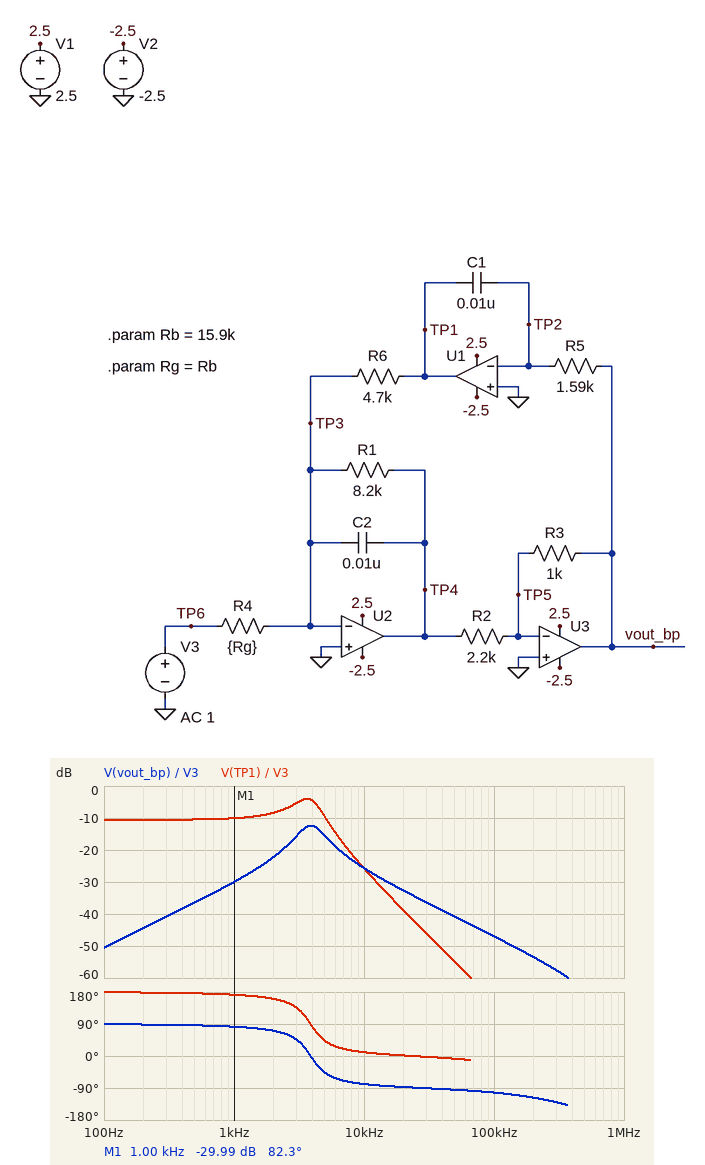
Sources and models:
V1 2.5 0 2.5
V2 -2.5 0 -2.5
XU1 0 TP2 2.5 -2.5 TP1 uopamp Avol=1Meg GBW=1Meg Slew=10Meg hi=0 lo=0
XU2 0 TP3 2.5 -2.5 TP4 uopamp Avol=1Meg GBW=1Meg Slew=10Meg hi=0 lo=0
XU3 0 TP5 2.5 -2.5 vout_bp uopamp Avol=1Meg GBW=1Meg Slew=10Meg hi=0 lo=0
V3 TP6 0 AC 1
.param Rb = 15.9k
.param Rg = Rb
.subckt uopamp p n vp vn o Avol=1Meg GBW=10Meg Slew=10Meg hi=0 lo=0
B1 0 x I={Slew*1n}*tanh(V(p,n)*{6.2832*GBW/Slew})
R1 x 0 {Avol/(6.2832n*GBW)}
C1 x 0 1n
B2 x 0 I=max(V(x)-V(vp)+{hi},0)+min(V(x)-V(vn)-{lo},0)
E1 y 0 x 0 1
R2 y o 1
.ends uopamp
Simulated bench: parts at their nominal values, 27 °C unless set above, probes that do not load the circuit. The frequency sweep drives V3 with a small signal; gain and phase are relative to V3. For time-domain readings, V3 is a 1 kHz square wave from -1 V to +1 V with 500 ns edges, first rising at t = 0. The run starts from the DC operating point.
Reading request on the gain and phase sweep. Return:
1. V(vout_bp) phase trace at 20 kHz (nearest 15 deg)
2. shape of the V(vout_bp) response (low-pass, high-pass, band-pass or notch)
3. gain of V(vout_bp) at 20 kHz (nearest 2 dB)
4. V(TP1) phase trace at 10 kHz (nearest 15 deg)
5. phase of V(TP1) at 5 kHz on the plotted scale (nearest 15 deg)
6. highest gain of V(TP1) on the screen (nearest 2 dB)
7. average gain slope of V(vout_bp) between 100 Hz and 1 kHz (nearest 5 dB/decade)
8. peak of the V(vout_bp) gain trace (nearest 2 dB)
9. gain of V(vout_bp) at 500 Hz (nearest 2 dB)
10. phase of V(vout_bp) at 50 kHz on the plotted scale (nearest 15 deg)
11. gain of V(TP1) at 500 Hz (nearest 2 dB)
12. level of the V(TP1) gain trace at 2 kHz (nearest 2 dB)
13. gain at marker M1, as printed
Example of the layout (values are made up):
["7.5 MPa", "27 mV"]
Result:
["-90 deg", "band-pass", "-32 dB", "15 deg", "45 deg", "-4 dB", "20 dB/decade", "-12 dB", "-36 dB", "-90 deg", "-10 dB", "-8 dB", "-29.99 dB"]
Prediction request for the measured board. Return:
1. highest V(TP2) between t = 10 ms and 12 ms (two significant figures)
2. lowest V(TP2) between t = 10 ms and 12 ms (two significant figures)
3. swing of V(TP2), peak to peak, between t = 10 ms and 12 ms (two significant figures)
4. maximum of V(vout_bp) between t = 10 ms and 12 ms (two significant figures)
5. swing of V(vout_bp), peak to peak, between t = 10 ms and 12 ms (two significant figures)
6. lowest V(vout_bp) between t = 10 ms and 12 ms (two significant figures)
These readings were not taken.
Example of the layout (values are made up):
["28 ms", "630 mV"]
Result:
["1.6 mV", "-1.6 mV", "3.2 mV", "160 mV", "320 mV", "-160 mV"]
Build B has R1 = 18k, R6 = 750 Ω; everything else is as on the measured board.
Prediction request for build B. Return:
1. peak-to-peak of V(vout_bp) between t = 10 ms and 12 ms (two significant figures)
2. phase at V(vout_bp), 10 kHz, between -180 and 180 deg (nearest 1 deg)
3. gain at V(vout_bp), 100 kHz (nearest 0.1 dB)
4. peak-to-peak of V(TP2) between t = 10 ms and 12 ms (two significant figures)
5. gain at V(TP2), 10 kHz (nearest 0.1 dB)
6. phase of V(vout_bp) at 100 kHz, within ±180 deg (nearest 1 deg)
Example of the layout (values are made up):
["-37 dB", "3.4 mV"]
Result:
["140 mV", "-52 deg", "-47.1 dB", "1.4 mV", "-45.7 dB", "-104 deg"]
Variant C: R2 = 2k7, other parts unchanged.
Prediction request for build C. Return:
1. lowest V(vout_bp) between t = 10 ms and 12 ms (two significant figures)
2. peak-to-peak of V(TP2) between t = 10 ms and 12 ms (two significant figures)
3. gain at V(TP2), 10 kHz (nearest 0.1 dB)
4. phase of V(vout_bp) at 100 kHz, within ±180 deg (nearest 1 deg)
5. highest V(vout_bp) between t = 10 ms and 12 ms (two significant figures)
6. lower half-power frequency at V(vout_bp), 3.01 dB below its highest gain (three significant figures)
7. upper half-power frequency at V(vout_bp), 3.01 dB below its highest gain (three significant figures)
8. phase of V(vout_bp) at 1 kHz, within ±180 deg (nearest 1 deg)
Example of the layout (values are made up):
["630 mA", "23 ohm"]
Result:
["-150 mV", "3.0 mV", "-67.8 dB", "-102 deg", "150 mV", "2.70 kHz", "4.59 kHz", "80 deg"]
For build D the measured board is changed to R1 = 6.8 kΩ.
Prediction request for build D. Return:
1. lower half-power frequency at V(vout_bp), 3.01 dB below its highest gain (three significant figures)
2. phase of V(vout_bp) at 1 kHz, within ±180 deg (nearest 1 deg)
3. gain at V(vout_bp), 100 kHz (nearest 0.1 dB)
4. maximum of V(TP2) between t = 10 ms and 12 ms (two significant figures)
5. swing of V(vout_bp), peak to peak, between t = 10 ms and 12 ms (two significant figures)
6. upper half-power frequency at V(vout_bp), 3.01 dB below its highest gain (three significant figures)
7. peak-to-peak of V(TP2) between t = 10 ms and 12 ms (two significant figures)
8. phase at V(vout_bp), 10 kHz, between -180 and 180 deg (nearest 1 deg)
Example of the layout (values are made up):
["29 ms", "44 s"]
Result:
["2.92 kHz", "81 deg", "-47.0 dB", "1.5 mV", "310 mV", "5.20 kHz", "3.1 mV", "-76 deg"]
